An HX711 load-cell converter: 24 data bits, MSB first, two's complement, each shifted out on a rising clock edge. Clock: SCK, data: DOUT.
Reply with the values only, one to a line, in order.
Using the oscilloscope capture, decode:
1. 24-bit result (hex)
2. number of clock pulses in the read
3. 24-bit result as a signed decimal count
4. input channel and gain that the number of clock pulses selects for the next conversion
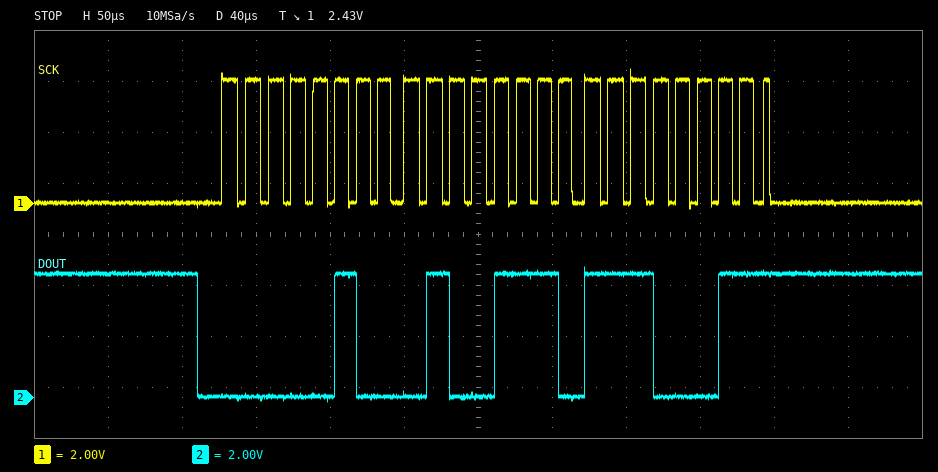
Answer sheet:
0x044EE3
25
282339
channel A, gain 128
